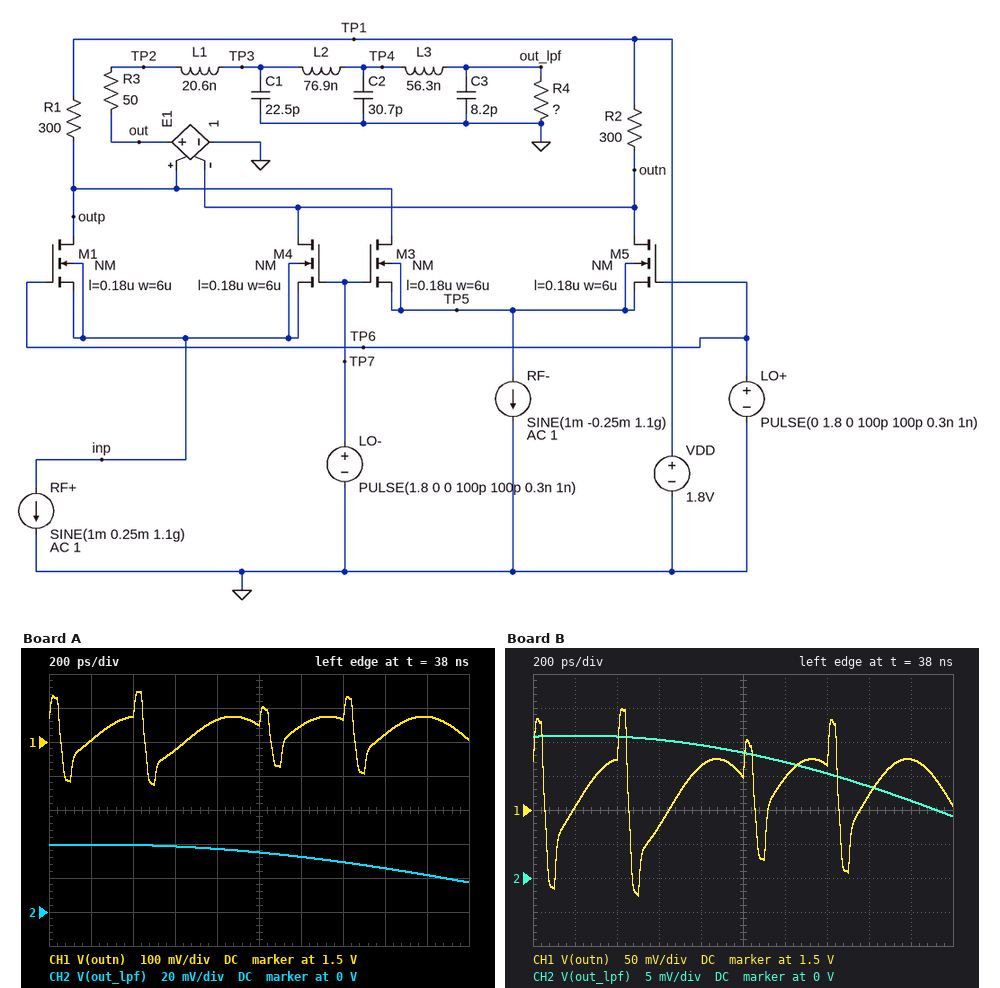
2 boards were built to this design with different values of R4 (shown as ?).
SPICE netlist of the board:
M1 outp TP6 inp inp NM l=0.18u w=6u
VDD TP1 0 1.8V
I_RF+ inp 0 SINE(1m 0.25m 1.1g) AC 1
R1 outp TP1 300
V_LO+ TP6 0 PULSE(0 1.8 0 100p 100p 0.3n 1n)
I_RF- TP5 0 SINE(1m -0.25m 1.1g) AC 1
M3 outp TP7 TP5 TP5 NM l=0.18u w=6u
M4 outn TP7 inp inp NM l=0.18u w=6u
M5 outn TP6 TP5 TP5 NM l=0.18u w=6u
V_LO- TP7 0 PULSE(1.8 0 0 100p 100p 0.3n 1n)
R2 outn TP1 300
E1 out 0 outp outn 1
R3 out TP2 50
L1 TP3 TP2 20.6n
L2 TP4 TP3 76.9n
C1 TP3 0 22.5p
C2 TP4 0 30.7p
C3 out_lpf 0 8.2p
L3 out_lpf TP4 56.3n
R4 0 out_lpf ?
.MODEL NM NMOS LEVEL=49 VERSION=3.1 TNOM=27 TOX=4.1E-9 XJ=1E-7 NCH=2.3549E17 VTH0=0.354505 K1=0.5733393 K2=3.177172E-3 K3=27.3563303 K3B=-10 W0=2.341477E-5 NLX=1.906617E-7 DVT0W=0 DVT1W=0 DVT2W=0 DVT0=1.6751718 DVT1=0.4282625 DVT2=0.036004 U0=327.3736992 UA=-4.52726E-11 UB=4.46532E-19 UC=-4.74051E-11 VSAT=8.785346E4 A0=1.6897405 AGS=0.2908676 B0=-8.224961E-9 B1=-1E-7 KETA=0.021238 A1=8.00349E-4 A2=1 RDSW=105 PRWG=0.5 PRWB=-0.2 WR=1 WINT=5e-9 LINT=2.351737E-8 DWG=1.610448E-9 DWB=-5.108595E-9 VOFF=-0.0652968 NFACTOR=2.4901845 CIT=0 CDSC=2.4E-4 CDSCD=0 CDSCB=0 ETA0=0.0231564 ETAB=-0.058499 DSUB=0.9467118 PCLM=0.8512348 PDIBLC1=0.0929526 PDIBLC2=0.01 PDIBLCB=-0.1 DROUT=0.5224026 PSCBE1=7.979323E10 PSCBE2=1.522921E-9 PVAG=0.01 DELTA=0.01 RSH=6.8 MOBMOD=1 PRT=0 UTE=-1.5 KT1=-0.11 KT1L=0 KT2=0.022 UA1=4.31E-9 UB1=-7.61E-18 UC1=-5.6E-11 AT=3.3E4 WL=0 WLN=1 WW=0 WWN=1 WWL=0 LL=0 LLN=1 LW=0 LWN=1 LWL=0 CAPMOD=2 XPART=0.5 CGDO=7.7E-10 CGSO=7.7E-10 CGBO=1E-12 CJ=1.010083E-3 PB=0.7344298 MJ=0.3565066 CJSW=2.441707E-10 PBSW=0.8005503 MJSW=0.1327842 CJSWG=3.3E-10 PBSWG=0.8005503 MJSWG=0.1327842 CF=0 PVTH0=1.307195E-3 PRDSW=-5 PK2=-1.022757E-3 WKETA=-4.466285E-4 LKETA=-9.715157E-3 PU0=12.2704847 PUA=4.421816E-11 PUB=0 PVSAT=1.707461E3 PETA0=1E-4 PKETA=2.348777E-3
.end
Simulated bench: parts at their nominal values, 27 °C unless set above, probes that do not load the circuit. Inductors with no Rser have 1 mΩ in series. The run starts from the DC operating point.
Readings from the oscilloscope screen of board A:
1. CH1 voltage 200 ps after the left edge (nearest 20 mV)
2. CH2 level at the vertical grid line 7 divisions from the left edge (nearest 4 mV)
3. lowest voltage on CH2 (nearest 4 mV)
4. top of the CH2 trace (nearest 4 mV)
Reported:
1.50 V
28 mV
16 mV
40 mV
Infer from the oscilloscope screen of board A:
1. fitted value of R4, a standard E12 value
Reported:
39 Ω
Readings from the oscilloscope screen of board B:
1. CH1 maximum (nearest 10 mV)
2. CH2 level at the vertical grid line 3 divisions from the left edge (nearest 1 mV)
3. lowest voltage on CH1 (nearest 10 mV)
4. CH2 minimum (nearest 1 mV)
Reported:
1.65 V
20 mV
1.37 V
9 mV
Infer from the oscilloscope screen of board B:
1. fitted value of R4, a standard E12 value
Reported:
15 Ω
